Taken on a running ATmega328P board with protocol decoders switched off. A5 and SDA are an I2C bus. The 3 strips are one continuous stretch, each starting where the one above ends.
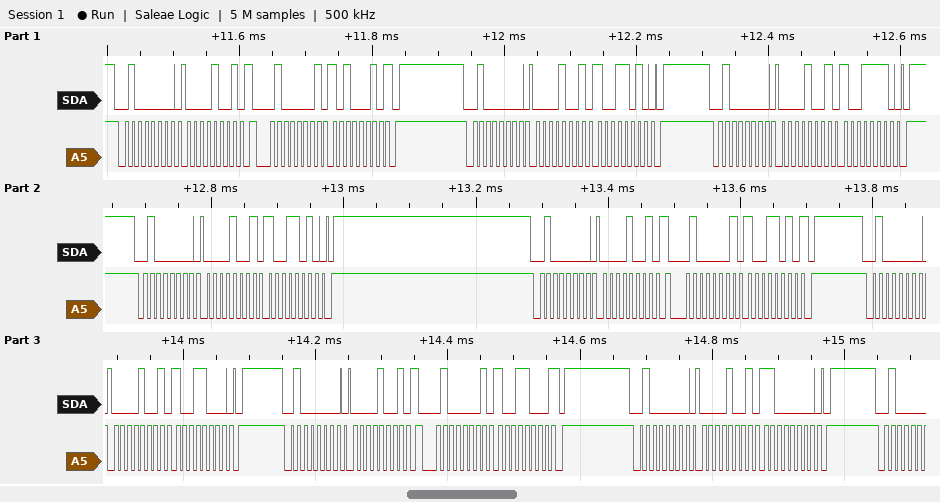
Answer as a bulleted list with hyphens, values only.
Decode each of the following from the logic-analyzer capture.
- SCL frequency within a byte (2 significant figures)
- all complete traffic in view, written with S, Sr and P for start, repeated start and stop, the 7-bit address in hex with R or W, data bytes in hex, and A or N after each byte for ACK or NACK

- 100 kHz
- S 20W A 09 A Sr 20R A A2 N P S 20W A 09 A 9A A P S 20W A 09 A 9E A P S 20W A 09 A 9A A P S 20W A 09 A Sr 20R A 9A N P S 20W A 09 A 98 A P S 20W A 09 A Sr 20R A 98 N P S 20W A 09 A C0 A P
